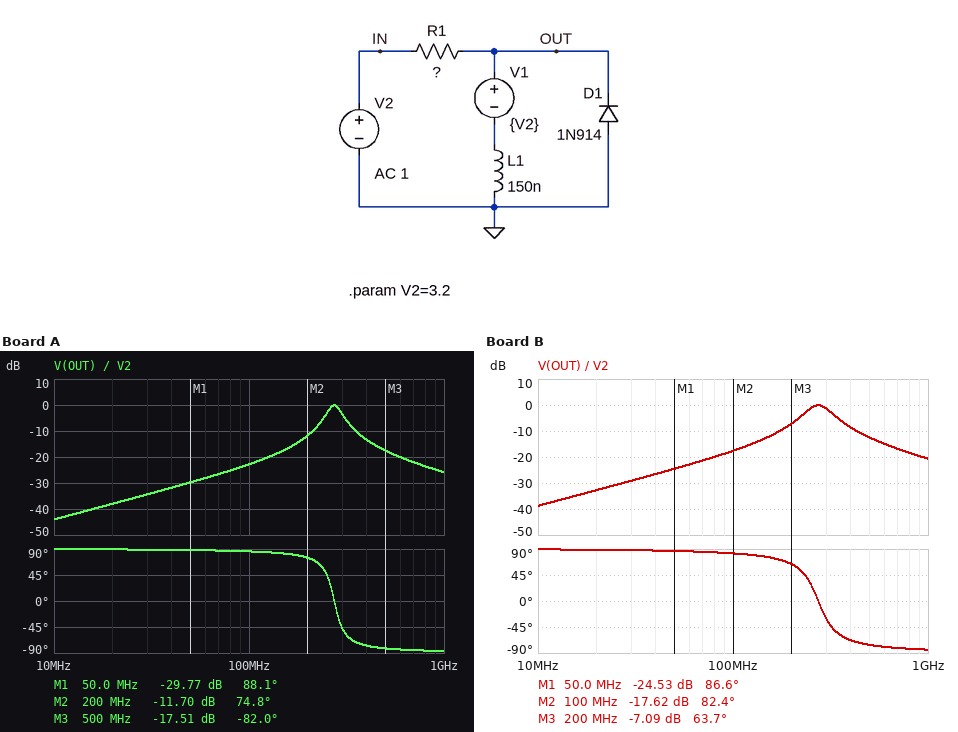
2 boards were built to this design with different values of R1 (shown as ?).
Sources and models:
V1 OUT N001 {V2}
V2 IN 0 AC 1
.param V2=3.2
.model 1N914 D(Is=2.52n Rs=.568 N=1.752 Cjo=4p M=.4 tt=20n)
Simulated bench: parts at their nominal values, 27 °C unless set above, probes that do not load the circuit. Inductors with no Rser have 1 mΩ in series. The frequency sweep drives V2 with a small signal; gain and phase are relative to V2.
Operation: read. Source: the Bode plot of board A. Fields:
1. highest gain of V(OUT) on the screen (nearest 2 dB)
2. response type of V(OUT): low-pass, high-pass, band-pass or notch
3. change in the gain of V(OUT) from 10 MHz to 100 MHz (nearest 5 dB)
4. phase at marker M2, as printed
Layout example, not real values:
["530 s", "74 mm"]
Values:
["0 dB", "band-pass", "20 dB", "74.8 deg"]
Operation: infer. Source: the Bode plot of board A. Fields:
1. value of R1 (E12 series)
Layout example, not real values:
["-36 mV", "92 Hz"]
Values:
["1.5 kΩ"]
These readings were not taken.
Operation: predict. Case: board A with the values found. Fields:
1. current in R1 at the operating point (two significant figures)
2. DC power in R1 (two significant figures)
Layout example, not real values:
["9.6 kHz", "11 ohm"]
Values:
["2.1 mA", "6.8 mW"]
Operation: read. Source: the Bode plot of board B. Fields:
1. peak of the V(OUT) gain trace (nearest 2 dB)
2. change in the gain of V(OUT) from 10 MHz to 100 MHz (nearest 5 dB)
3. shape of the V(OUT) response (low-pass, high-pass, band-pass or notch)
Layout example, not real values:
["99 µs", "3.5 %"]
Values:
["0 dB", "20 dB", "band-pass"]
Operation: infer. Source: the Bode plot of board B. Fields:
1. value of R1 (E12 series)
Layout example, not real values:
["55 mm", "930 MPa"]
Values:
["820 Ω"]
